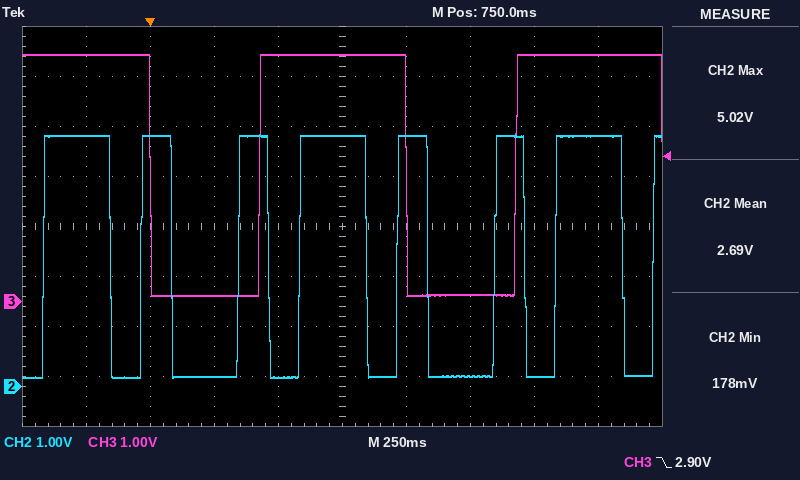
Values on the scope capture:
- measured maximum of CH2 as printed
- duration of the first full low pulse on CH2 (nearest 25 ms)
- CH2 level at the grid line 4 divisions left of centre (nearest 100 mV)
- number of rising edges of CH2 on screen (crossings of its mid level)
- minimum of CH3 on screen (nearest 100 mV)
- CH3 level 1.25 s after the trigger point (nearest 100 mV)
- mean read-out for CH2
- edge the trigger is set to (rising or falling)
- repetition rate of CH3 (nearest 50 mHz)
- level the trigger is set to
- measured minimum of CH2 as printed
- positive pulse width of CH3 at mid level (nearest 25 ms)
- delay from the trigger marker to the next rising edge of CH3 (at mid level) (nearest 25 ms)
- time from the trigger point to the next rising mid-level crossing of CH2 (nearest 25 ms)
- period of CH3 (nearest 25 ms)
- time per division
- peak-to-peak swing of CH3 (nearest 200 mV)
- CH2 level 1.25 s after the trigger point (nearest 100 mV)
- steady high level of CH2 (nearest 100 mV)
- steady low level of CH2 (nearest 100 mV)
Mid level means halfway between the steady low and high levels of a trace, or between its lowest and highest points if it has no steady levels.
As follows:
5.02 V
125 ms
5.0 V
8
100 mV
100 mV
2.69 V
falling
1.00 Hz
2.90 V
178 mV
575 ms
425 ms
350 ms
1.000 s
250 ms
4.8 V
200 mV
5.0 V
200 mV
